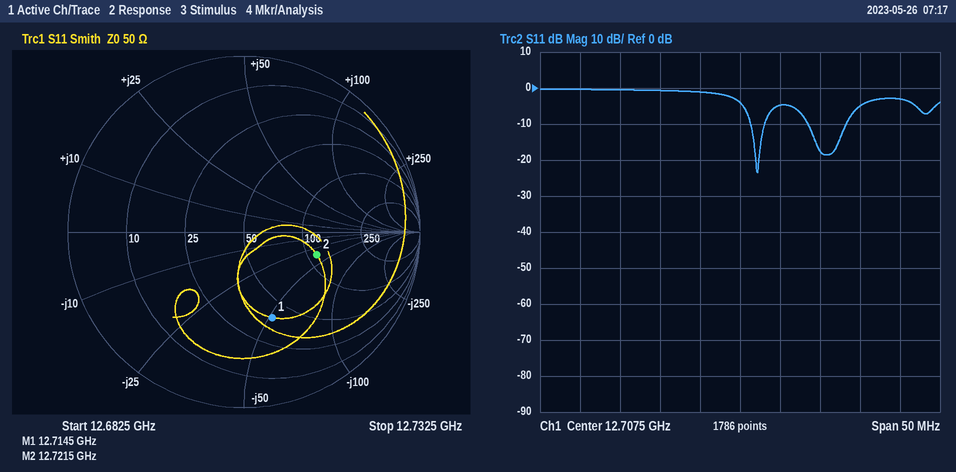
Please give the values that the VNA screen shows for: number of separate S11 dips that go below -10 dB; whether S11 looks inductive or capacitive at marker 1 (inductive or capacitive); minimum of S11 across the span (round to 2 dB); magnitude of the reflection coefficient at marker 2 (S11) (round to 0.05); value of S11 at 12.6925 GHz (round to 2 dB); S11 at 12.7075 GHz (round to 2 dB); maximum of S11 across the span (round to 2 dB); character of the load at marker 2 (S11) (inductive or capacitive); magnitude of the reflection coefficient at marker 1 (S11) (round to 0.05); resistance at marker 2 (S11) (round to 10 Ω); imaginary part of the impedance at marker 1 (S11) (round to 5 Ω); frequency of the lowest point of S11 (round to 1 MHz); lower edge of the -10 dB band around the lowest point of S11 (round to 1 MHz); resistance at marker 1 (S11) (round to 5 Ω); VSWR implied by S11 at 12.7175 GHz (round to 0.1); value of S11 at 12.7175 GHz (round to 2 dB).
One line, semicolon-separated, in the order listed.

2; capacitive; -24 dB; 0.45; 0 dB; -4 dB; 0 dB; capacitive; 0.50; 110 Ω; -50 Ω; 12.710 GHz; 12.709 GHz; 40 Ω; 1.3; -18 dB
